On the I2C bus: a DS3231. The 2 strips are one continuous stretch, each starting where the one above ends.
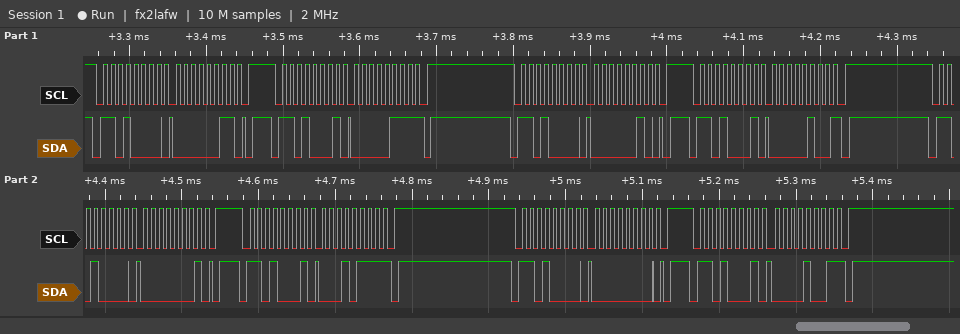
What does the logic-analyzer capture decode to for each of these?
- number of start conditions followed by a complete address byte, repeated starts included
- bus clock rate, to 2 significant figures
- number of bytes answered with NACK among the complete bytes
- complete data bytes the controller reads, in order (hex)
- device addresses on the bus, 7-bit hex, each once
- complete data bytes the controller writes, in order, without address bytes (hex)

8
100 kHz
4
07 04 17 09
0x68
03 02 01 00
